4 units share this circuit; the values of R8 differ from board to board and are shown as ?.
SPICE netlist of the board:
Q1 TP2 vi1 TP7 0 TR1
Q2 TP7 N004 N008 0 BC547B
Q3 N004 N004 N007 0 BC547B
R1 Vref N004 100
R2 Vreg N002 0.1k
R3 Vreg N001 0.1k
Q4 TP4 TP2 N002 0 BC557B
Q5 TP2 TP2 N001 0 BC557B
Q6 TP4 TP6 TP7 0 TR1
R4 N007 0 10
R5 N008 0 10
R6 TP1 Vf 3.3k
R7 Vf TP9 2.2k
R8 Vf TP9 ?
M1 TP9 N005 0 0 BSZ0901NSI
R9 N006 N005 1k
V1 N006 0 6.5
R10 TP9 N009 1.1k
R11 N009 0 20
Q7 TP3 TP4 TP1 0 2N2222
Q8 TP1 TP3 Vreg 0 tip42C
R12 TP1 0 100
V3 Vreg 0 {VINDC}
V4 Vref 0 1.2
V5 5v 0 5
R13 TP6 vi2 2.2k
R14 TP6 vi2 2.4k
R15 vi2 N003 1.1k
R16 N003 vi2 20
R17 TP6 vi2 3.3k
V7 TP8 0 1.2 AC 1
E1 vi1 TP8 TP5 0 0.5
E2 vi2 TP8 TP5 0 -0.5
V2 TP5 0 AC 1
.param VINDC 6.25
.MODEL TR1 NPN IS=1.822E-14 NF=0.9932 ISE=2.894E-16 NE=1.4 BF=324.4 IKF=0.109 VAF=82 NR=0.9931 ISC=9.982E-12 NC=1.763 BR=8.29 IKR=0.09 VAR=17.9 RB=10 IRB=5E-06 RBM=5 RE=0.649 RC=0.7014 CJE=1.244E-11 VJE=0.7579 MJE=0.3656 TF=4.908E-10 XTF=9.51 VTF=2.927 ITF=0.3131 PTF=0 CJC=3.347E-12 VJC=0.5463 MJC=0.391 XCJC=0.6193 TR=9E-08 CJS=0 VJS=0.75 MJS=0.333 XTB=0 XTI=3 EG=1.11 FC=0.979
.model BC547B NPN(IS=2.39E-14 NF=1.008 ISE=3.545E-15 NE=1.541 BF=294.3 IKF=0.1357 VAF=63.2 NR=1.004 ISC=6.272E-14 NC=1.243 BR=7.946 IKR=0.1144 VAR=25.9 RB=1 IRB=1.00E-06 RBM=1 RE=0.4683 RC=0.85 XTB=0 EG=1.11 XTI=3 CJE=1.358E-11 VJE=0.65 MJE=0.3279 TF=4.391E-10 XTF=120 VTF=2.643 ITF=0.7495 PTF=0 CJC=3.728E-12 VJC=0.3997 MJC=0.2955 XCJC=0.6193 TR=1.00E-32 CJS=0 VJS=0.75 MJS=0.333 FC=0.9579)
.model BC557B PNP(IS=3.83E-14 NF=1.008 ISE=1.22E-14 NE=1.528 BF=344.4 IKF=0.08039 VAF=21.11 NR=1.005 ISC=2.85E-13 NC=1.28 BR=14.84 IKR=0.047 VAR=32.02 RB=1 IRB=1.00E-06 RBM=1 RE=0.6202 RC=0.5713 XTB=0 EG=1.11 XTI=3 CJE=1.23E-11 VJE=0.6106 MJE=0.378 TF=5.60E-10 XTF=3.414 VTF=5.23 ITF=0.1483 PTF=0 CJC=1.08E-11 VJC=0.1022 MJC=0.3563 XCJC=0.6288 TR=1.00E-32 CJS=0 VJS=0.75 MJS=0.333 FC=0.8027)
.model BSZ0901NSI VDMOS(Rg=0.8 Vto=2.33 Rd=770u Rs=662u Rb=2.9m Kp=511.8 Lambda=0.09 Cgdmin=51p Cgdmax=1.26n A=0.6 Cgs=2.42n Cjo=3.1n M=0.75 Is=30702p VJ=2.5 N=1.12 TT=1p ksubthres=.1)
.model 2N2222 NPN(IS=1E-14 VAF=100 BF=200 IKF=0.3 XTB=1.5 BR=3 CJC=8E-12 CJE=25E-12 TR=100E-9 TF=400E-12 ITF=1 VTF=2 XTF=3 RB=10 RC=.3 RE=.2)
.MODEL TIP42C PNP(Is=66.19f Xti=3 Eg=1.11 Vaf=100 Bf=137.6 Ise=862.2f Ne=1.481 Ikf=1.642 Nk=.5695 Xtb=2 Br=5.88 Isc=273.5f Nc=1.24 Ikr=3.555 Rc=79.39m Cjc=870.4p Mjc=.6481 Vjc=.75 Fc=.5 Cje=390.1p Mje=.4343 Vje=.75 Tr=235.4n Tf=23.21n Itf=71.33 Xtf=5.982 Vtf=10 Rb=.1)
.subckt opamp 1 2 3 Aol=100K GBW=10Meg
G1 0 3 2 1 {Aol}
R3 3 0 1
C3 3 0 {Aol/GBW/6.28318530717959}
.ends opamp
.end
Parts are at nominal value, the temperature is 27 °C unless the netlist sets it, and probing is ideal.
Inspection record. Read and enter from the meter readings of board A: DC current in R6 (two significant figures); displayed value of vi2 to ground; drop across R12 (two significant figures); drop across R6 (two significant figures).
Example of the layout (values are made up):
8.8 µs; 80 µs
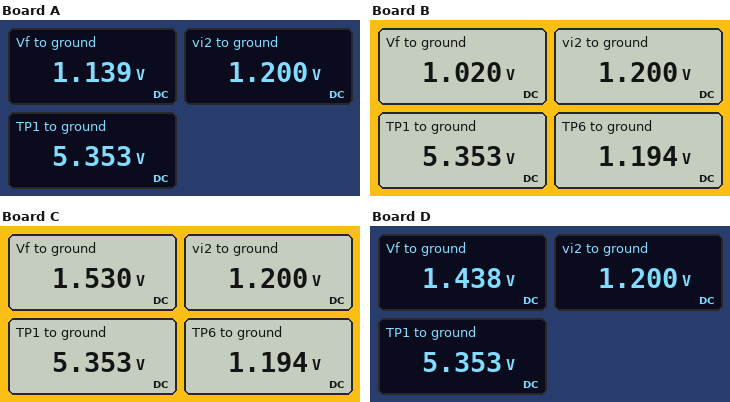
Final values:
1.3 mA; 1.200 V; 5.4 V; 4.2 V
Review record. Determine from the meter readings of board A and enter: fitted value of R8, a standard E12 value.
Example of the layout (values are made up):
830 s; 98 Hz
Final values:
1.5 kΩ
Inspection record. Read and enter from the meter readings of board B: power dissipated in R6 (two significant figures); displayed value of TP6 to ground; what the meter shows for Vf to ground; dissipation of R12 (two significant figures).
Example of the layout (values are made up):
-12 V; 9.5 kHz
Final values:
5.7 mW; 1.194 V; 1.020 V; 290 mW
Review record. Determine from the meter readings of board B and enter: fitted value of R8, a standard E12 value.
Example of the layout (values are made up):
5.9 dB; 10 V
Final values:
1.2 kΩ
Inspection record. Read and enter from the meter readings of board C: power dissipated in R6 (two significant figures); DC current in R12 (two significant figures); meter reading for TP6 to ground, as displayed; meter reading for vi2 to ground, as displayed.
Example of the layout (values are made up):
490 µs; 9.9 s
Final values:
4.4 mW; 54 mA; 1.194 V; 1.200 V
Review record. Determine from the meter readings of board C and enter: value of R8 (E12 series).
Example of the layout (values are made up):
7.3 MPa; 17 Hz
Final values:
3.3 kΩ
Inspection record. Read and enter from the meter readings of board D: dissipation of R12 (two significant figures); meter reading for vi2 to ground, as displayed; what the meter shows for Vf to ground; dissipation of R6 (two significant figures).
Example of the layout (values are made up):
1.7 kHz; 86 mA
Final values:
290 mW; 1.200 V; 1.438 V; 4.6 mW
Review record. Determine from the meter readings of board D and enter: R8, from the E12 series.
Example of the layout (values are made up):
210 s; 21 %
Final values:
2.7 kΩ
